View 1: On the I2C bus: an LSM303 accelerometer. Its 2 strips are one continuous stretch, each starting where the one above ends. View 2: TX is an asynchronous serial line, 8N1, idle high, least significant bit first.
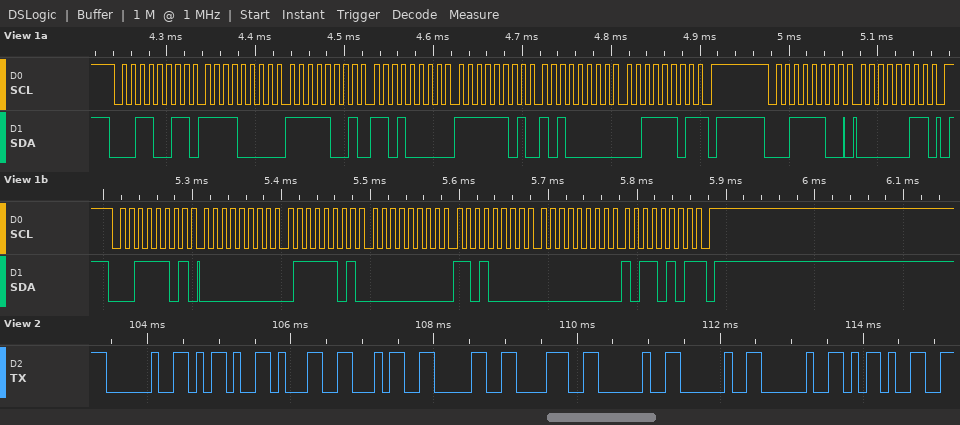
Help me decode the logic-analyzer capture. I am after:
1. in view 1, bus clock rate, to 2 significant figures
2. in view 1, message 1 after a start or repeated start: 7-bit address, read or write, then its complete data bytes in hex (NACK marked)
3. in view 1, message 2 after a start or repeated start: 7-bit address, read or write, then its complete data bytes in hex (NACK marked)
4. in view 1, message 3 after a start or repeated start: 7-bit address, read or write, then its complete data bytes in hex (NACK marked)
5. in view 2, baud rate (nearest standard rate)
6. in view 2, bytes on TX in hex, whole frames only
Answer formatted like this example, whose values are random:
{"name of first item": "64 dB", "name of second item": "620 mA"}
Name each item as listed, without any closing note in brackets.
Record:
{"in view 1, bus clock rate, to 2 significant figures": "100 kHz", "in view 1, message 1 after a start or repeated start: 7-bit address, read or write, then its complete data bytes in hex": "0x19 read: F0 F9 D0 FD A0 3D NACK", "in view 1, message 2 after a start or repeated start: 7-bit address, read or write, then its complete data bytes in hex": "0x1E write: 03", "in view 1, message 3 after a start or repeated start: 7-bit address, read or write, then its complete data bytes in hex": "0x1E read: 00 7D 00 D0 00 B5 NACK", "in view 2, baud rate": "9600 baud", "in view 2, bytes on TX in hex, whole frames only": "20 2D 31 34 30 38 20 20 20 2D"}
